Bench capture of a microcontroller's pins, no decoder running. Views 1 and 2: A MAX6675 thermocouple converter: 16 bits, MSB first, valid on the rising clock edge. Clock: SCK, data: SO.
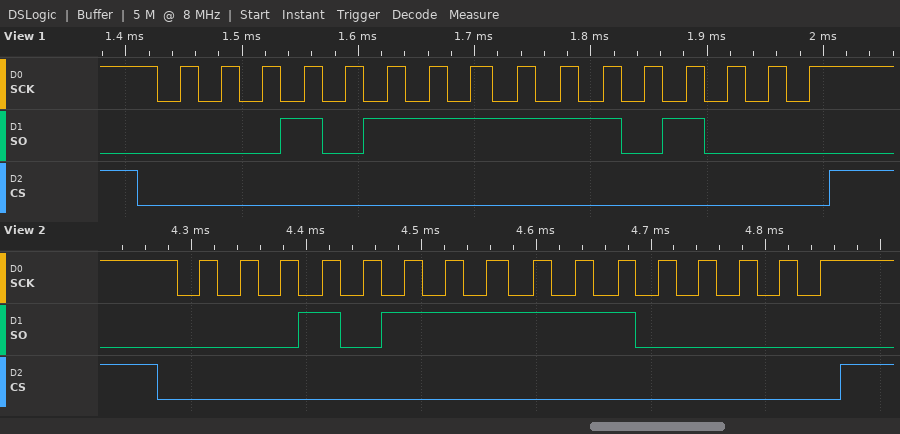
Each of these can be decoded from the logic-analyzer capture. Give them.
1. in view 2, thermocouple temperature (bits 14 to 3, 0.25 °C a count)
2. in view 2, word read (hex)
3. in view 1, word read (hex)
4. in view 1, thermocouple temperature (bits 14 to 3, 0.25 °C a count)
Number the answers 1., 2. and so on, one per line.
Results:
1. 191.00 °C
2. 0x17E0
3. 0x17E8
4. 191.25 °C
